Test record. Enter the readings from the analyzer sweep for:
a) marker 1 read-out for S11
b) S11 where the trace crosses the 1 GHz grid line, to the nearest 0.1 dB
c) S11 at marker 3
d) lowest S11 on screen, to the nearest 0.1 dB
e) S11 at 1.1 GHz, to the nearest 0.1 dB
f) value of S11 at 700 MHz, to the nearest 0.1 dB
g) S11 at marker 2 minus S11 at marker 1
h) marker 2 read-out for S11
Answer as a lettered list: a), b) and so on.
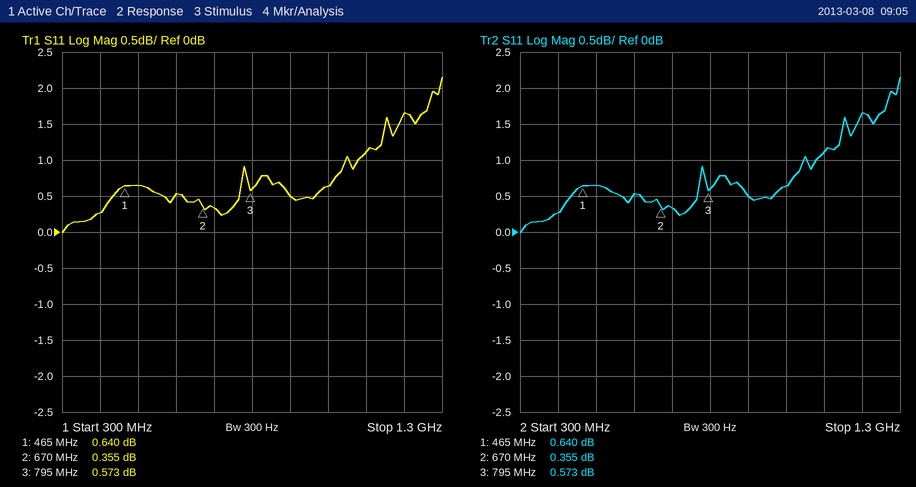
a) 0.640 dB
b) 0.6 dB
c) 0.573 dB
d) 0.0 dB
e) 1.1 dB
f) 0.3 dB
g) -0.285 dB
h) 0.355 dB
